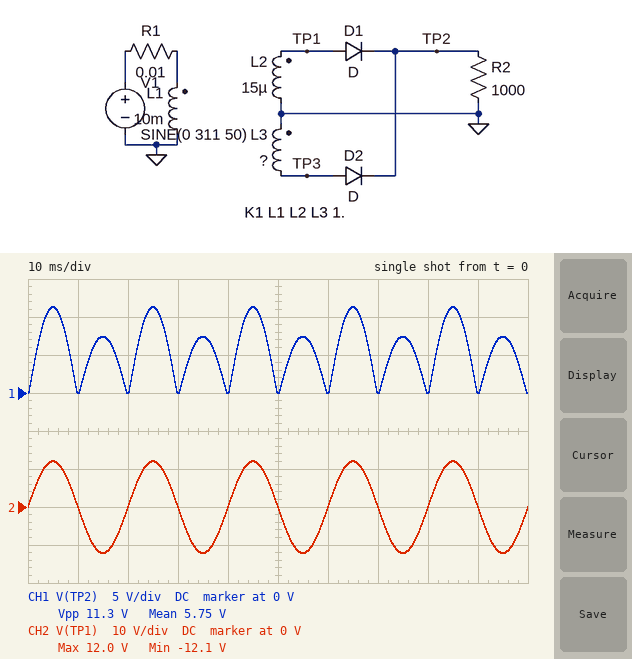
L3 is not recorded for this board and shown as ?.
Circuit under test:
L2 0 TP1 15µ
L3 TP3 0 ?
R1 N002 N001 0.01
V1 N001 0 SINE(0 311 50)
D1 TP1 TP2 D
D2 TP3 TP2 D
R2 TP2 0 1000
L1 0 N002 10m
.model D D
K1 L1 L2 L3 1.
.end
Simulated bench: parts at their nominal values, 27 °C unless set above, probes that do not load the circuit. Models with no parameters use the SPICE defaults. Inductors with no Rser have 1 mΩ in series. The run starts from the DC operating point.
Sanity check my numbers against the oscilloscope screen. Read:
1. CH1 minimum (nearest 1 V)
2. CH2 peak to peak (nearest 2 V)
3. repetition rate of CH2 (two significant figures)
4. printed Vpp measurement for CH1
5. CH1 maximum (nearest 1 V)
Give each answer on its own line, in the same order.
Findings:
0 V
24 V
50 Hz
11.3 V
11 V
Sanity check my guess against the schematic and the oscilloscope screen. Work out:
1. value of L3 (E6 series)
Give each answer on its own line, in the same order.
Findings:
6.8 µH
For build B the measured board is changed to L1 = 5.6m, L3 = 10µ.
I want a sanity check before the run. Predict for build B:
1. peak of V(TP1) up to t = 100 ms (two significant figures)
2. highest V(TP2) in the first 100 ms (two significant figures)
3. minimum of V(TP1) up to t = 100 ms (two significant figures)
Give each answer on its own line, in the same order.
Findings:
16 V
15 V
-16 V
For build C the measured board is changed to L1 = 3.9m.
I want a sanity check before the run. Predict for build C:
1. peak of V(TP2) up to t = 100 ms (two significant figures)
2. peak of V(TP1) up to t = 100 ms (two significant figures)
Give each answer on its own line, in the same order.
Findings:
18 V
19 V
